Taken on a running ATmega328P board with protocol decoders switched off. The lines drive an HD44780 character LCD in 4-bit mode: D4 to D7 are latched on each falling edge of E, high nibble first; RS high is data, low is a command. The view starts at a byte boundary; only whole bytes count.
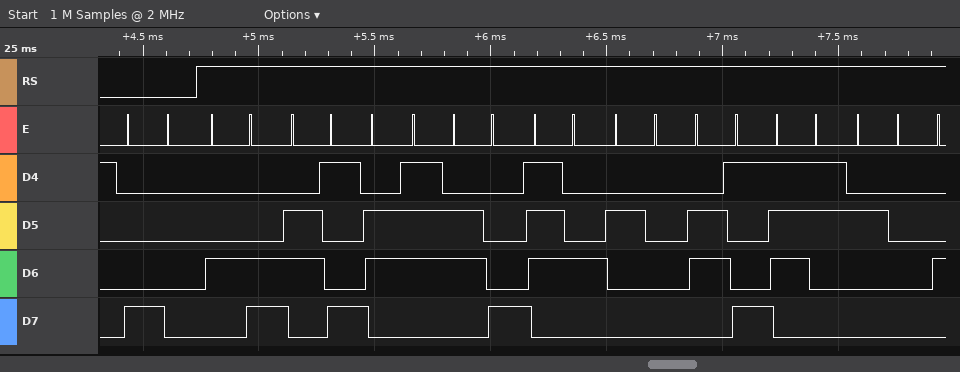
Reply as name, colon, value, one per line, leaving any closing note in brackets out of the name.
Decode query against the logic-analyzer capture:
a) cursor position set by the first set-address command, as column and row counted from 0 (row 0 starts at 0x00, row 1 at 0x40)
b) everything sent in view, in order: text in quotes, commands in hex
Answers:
cursor position set by the first set-address command, as column and row counted from 0: column 0, row 0
everything sent in view, in order: text in quotes, commands in hex: 0x80 "Light is "
